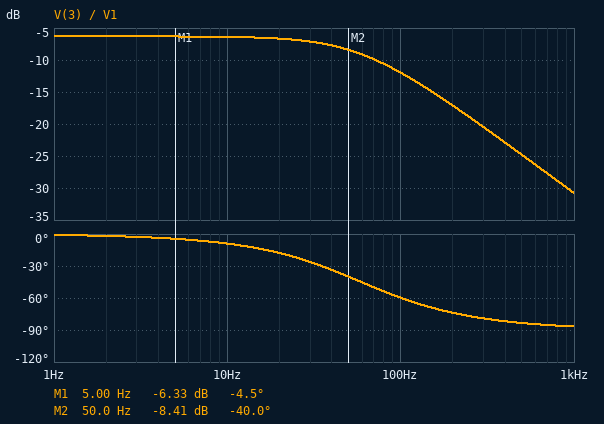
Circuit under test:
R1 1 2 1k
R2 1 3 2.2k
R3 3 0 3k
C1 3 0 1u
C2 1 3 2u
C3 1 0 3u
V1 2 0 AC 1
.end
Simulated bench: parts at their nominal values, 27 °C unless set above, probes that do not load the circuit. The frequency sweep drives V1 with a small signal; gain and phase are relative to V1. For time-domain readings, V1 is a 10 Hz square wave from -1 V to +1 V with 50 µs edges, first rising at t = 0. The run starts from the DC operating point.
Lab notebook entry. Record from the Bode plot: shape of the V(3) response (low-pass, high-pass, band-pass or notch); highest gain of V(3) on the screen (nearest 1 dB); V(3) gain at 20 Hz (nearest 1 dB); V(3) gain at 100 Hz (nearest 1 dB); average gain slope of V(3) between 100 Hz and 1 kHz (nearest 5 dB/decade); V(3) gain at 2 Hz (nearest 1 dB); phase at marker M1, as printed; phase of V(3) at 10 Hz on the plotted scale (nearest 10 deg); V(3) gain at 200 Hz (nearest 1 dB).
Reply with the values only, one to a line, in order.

low-pass
-6 dB
-7 dB
-12 dB
-20 dB/decade
-6 dB
-4.5 deg
-10 deg
-17 dB
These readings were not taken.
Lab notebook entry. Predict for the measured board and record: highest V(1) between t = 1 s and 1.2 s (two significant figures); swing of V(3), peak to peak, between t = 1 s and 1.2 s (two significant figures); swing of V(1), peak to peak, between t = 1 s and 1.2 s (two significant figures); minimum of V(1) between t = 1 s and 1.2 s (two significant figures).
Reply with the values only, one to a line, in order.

840 mV
970 mV
1.7 V
-840 mV
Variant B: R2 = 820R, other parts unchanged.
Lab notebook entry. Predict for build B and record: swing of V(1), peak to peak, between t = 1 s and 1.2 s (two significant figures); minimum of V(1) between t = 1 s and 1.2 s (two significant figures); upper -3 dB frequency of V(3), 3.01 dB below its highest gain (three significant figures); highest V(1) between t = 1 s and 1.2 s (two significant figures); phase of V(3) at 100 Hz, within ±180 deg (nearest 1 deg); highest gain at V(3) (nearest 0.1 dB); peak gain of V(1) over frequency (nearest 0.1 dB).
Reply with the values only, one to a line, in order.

1.6 V
-790 mV
49.8 Hz
790 mV
-66 deg
-4.1 dB
-2.0 dB
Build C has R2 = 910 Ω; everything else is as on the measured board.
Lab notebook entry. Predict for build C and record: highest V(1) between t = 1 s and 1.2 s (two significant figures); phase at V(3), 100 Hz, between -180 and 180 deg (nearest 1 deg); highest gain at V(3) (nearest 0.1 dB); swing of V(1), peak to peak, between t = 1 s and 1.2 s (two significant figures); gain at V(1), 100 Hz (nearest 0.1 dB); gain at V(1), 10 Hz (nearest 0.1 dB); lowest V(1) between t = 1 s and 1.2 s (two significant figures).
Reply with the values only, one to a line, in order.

800 mV
-65 deg
-4.3 dB
1.6 V
-8.4 dB
-2.1 dB
-800 mV
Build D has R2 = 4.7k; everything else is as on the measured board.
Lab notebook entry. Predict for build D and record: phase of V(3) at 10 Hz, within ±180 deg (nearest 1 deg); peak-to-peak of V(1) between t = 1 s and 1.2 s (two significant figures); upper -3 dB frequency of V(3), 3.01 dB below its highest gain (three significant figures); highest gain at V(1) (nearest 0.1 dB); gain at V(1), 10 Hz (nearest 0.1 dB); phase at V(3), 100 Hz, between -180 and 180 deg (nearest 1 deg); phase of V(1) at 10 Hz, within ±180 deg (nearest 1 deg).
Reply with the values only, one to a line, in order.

-1 deg
1.8 V
81.8 Hz
-1.1 dB
-1.3 dB
-57 deg
-12 deg
